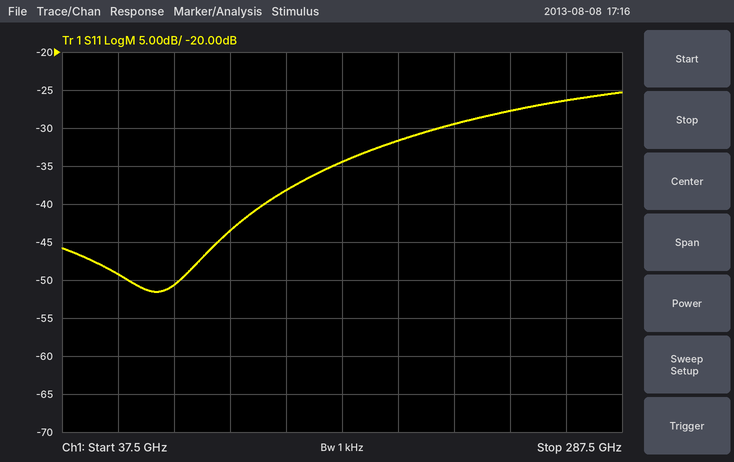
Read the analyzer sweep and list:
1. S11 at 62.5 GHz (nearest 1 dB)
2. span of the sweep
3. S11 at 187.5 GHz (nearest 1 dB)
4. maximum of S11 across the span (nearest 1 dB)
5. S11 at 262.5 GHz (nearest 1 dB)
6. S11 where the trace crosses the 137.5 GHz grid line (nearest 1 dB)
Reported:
-49 dB
250 GHz
-32 dB
-25 dB
-26 dB
-38 dB
